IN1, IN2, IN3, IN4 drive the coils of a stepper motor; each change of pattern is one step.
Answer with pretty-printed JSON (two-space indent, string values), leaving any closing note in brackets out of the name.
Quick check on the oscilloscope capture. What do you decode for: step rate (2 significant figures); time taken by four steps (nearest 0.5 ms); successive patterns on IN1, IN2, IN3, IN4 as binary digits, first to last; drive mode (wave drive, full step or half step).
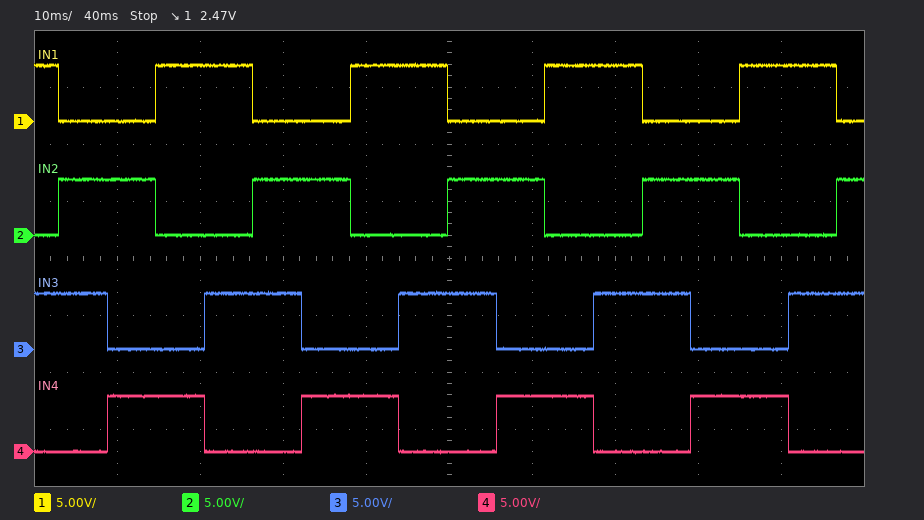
{
  "step rate": "170 steps/s",
  "time taken by four steps": "23.5 ms",
  "successive patterns on IN1, IN2, IN3, IN4 as binary digits, first to last": "1010 0110 0101 1001 1010 0110 0101 1001 1010 0110 0101 1001 1010 0110 0101 1001 1010 0110",
  "drive mode": "full step"
}
